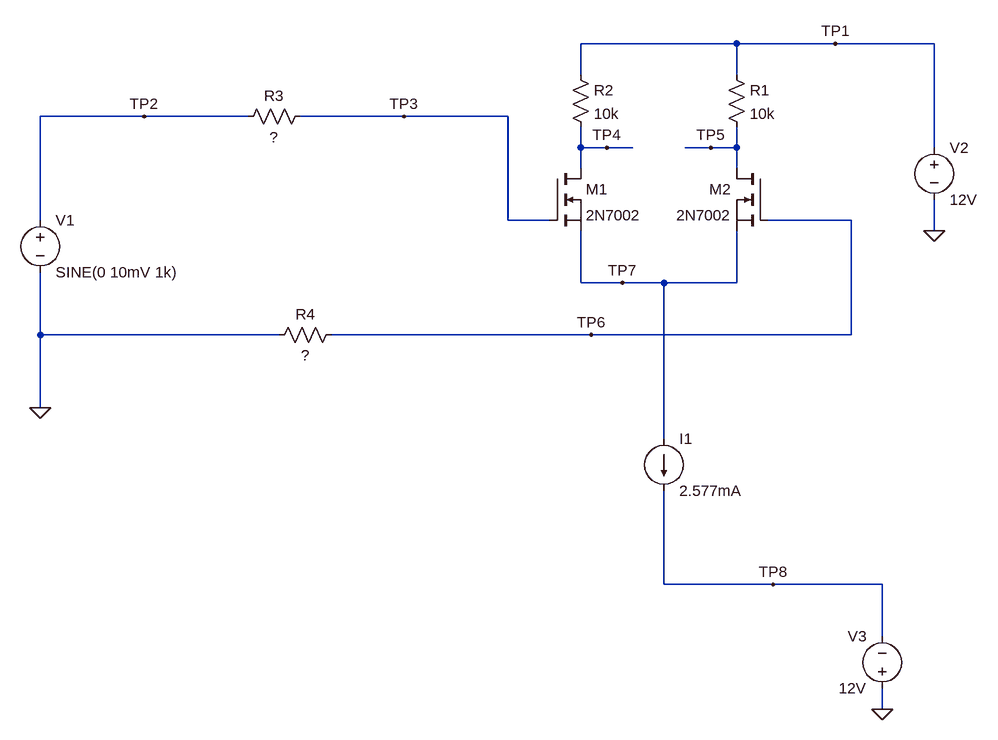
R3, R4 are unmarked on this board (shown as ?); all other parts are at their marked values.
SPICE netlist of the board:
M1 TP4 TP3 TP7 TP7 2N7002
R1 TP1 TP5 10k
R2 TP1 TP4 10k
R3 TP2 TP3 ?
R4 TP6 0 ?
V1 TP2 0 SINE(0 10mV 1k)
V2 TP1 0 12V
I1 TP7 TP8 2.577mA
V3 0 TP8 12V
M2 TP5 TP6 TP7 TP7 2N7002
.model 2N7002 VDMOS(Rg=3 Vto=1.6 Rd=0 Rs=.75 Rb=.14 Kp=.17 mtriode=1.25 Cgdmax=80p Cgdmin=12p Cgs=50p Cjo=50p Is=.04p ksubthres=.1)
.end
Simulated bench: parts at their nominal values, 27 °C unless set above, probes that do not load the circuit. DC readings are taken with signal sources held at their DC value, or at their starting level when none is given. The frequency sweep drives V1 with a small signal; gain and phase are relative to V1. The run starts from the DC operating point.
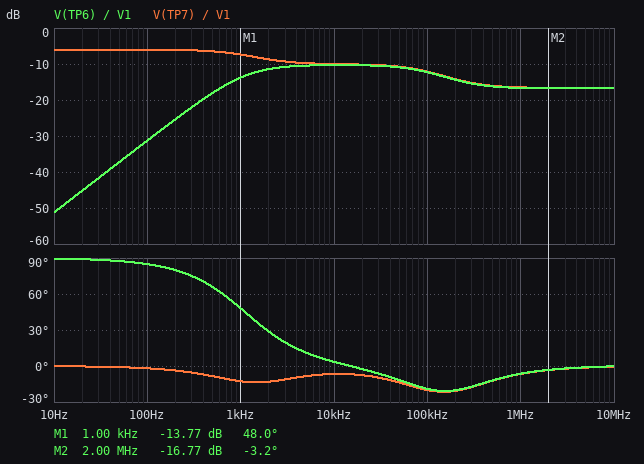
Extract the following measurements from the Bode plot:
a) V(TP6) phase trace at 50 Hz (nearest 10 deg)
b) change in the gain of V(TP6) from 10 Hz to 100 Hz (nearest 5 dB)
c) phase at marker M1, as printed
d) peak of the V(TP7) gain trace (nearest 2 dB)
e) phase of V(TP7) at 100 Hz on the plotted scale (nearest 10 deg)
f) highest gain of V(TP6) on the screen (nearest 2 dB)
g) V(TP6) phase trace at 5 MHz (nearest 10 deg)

90 deg
20 dB
48.0 deg
-6 dB
0 deg
-10 dB
0 deg
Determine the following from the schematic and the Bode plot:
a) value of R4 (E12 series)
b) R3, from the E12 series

8.2 kΩ
18 kΩ
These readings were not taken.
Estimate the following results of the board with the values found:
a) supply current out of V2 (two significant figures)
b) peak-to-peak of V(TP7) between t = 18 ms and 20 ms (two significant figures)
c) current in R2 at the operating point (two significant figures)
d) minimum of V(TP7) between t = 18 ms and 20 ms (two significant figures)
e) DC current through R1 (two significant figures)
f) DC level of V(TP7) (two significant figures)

2.6 mA
8.6 mV
1.3 mA
-1.7 V
1.3 mA
-1.7 V
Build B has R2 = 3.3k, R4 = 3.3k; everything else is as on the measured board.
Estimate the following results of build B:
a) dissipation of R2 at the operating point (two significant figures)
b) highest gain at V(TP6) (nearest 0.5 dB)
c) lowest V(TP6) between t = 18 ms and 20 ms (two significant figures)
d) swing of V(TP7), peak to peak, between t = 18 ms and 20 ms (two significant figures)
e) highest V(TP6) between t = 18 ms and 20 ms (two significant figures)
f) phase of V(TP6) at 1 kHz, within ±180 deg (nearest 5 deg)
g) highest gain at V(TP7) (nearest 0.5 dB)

5.5 mW
-3.5 dB
-1.1 mV
10 mV
1.1 mV
80 deg
-3.0 dB
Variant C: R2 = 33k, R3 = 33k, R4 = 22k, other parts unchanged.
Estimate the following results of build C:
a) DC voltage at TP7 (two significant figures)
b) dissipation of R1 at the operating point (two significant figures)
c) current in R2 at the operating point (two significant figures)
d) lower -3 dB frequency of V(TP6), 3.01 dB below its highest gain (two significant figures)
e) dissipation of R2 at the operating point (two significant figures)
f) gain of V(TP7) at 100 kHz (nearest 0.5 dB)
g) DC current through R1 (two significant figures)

-7.8 V
39 mW
600 µA
59 kHz
12 mW
-16.5 dB
2.0 mA
